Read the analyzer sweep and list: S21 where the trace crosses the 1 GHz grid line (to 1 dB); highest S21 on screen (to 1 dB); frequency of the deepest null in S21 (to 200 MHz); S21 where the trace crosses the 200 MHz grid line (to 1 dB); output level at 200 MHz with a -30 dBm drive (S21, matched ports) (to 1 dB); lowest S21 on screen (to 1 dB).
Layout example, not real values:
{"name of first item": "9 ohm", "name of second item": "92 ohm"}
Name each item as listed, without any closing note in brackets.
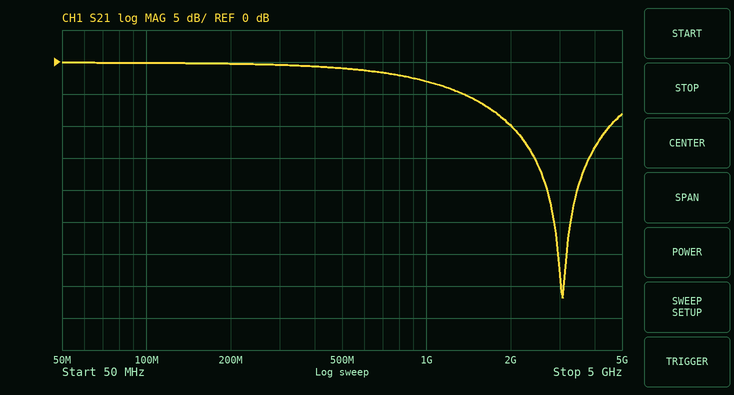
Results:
{"S21 where the trace crosses the 1 GHz grid line": "-3 dB", "highest S21 on screen": "0 dB", "frequency of the deepest null in S21": "3.0 GHz", "S21 where the trace crosses the 200 MHz grid line": "0 dB", "output level at 200 MHz with a -30 dBm drive (S21, matched ports)": "-30 dBm", "lowest S21 on screen": "-37 dB"}
